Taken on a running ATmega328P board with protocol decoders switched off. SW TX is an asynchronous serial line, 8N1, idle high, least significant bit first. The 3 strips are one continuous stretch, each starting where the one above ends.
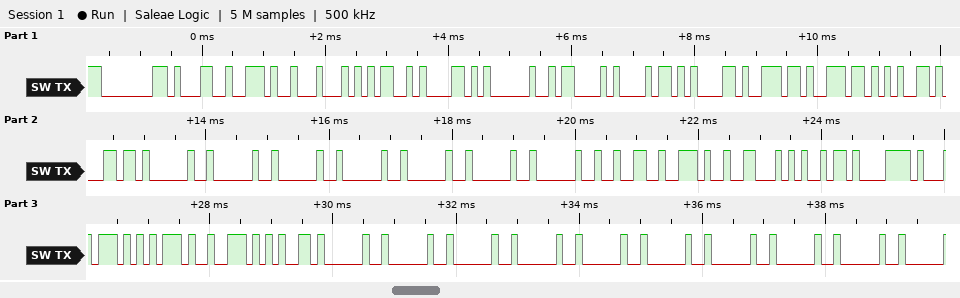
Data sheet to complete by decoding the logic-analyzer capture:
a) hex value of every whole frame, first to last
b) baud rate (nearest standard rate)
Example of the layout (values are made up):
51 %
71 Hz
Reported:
80 31 2E 44 4D 58 20 43 68 61 6E 6E 65 6C 20 20 20 20 20 20 20 32 2E 46 69 78 74 75 72 65 20 20 20 20 20 20 20 20 20
9600 baud
